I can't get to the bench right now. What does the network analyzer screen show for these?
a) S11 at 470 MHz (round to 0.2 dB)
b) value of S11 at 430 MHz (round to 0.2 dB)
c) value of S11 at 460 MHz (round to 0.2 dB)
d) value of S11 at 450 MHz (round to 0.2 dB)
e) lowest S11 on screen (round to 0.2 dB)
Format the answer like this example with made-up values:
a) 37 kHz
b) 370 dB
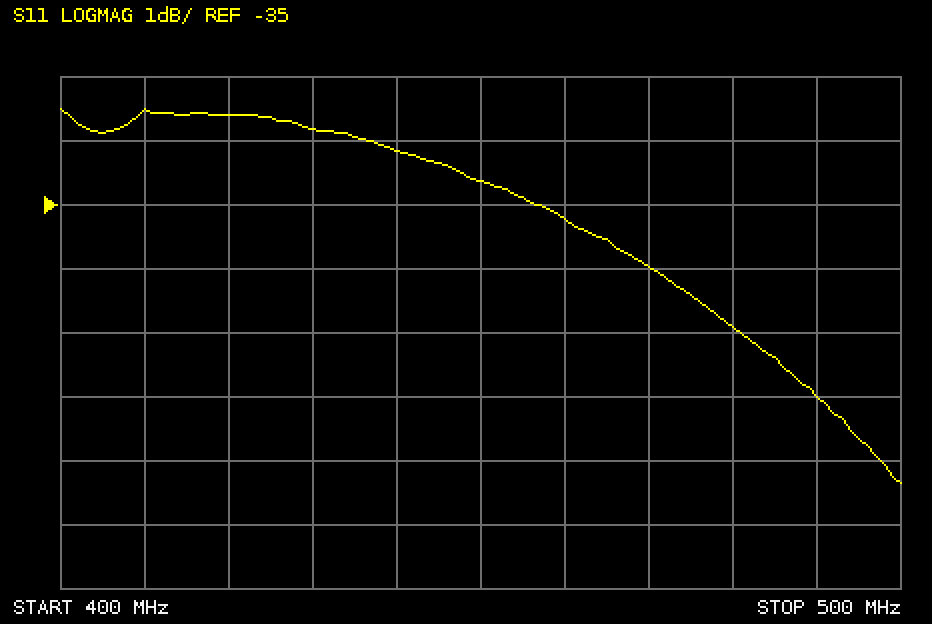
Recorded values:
a) -36.0 dB
b) -33.8 dB
c) -35.2 dB
d) -34.6 dB
e) -39.4 dB
